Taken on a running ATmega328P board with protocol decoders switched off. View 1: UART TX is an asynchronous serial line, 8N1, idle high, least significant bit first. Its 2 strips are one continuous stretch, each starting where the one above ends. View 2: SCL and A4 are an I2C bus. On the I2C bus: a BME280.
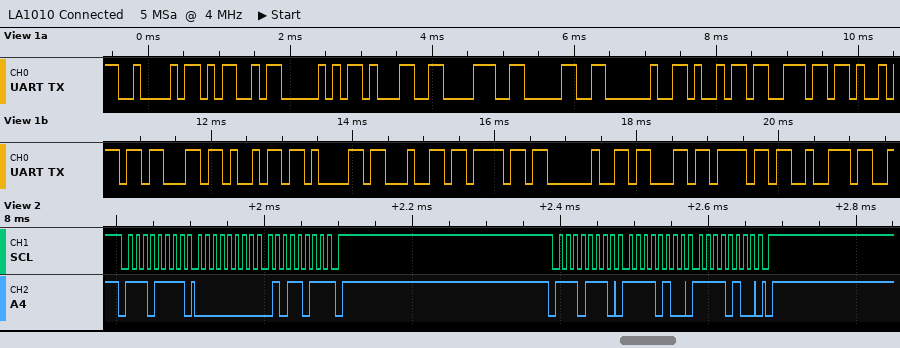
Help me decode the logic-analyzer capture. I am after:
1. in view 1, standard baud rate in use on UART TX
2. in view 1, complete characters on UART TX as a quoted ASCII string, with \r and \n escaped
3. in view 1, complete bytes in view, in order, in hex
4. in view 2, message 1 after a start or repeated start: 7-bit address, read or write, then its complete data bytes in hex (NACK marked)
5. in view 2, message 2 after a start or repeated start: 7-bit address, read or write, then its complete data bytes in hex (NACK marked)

9600 baud
"BMP180 iniciado cor"
0x42 0x4D 0x50 0x31 0x38 0x30 0x20 0x69 0x6E 0x69 0x63 0x69 0x61 0x64 0x6F 0x20 0x63 0x6F 0x72
0x77 read: 00 5B NACK
0x77 write: F4 F4
